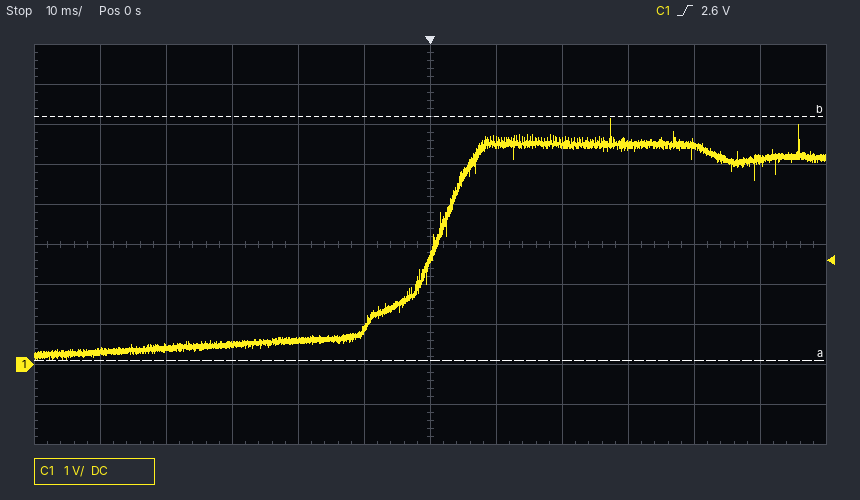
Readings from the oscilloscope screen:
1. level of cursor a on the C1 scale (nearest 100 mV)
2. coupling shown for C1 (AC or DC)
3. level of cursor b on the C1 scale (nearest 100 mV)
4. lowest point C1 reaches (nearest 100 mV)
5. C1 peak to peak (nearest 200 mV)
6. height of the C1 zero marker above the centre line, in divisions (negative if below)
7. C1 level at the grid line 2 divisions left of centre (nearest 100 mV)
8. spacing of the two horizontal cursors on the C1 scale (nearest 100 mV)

100 mV
DC
6.2 V
100 mV
6.0 V
-3.0 div
600 mV
6.1 V
